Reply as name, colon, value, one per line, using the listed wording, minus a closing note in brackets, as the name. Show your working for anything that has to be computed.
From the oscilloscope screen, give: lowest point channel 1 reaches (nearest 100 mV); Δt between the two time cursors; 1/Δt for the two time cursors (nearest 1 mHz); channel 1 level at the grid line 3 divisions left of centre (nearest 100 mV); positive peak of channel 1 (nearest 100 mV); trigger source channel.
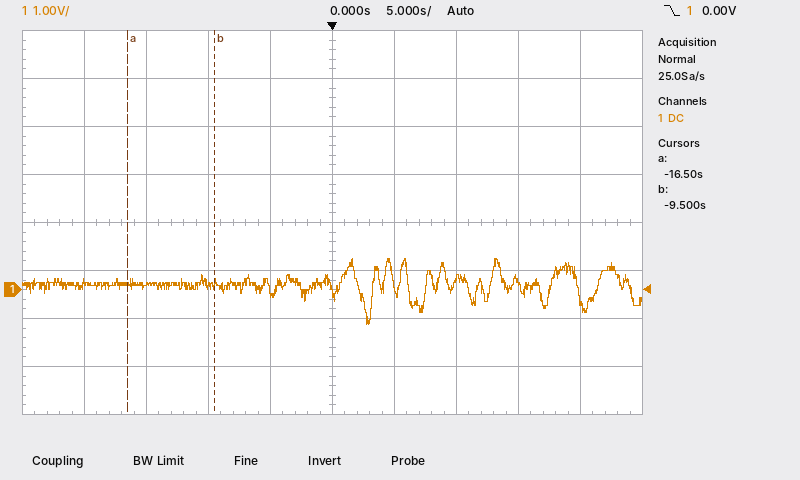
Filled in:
lowest point channel 1 reaches: -700 mV
Δt between the two time cursors: -9.5 s − (-16.5 s) = 7.0 s
1/Δt for the two time cursors: 1 / 7.0 s ≈ 143 mHz
channel 1 level at the grid line 3 divisions left of centre: 100 mV
positive peak of channel 1: 600 mV
trigger source channel: channel 1
